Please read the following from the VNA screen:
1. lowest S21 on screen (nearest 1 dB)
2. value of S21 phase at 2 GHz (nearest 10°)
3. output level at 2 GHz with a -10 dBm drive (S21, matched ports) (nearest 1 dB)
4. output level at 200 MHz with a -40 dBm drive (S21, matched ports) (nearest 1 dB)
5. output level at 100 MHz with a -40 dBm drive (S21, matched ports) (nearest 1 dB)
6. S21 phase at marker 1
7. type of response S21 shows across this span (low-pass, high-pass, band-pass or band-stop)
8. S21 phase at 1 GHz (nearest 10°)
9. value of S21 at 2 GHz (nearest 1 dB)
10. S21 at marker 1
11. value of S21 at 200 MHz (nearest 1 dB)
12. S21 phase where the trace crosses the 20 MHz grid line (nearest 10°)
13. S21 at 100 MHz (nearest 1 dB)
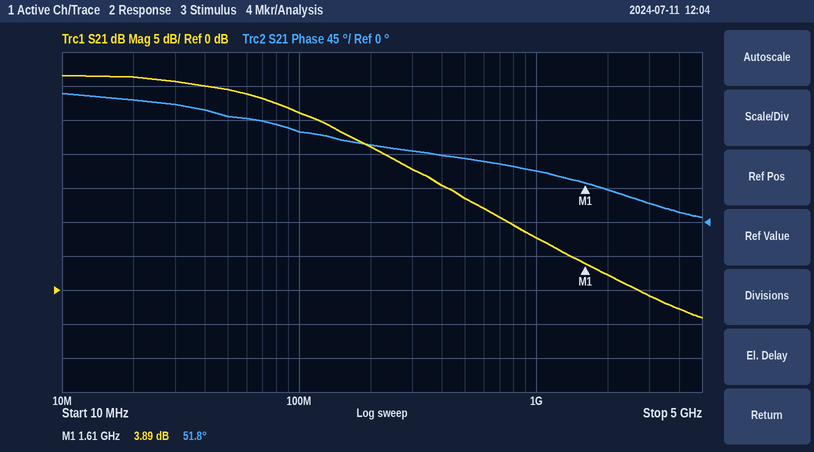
-4 dB
40°
-8 dBm
-19 dBm
-14 dBm
51.8°
low-pass
70°
2 dB
3.89 dB
21 dB
160°
26 dB
